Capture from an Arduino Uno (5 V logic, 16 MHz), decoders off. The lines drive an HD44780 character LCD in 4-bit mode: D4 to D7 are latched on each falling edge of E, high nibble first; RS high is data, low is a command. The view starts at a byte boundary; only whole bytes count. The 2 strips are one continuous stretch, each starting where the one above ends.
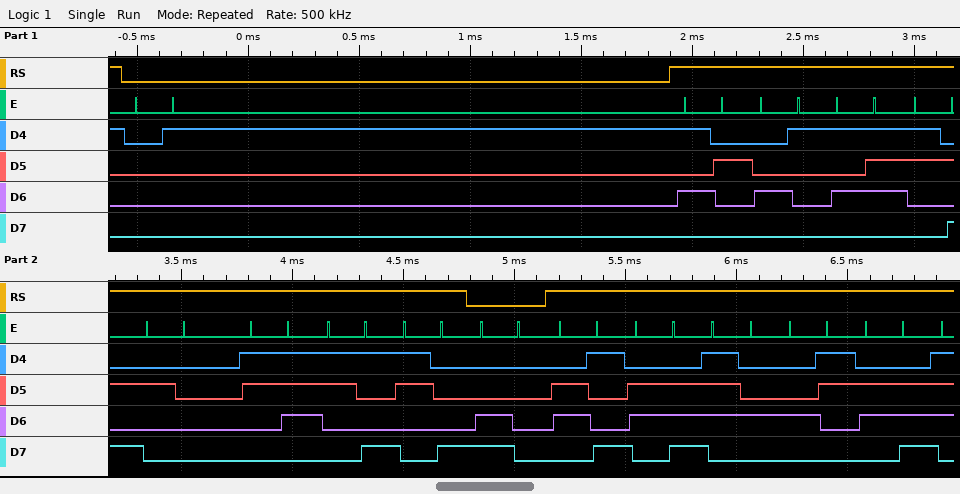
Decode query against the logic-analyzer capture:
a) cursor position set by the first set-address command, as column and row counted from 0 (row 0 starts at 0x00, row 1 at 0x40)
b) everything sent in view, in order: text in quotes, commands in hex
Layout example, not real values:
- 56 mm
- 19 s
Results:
- column 0, row 1
- 0x01 "RAW: 798" 0xC0 "intCn"
